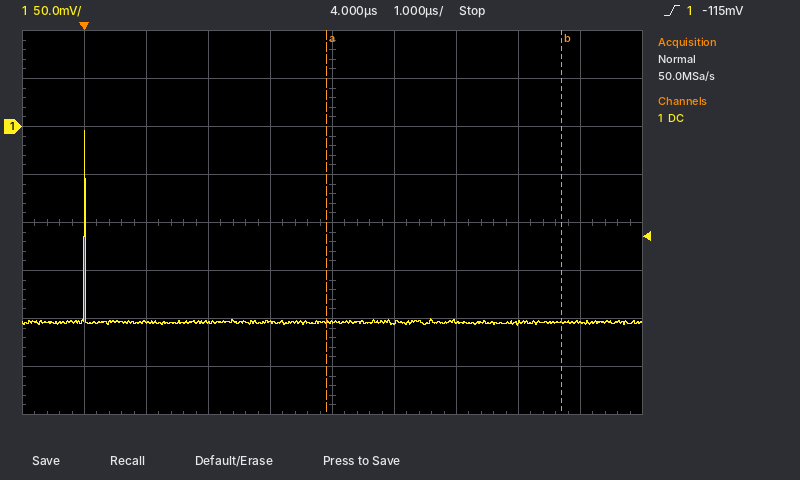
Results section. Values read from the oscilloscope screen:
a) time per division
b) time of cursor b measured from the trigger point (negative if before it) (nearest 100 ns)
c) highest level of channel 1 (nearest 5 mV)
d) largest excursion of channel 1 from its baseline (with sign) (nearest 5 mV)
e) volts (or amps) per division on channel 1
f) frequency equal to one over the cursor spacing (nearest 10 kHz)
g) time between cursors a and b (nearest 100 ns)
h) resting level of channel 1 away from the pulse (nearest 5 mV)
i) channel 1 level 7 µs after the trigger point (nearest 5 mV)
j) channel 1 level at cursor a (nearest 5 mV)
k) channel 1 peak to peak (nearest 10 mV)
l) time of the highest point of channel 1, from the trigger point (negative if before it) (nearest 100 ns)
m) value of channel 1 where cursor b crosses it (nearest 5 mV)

1 µs
+7.7 µs
-5 mV
+200 mV
50 mV
260 kHz
3.8 µs
-205 mV
-205 mV
-205 mV
200 mV
0.0 µs
-205 mV
